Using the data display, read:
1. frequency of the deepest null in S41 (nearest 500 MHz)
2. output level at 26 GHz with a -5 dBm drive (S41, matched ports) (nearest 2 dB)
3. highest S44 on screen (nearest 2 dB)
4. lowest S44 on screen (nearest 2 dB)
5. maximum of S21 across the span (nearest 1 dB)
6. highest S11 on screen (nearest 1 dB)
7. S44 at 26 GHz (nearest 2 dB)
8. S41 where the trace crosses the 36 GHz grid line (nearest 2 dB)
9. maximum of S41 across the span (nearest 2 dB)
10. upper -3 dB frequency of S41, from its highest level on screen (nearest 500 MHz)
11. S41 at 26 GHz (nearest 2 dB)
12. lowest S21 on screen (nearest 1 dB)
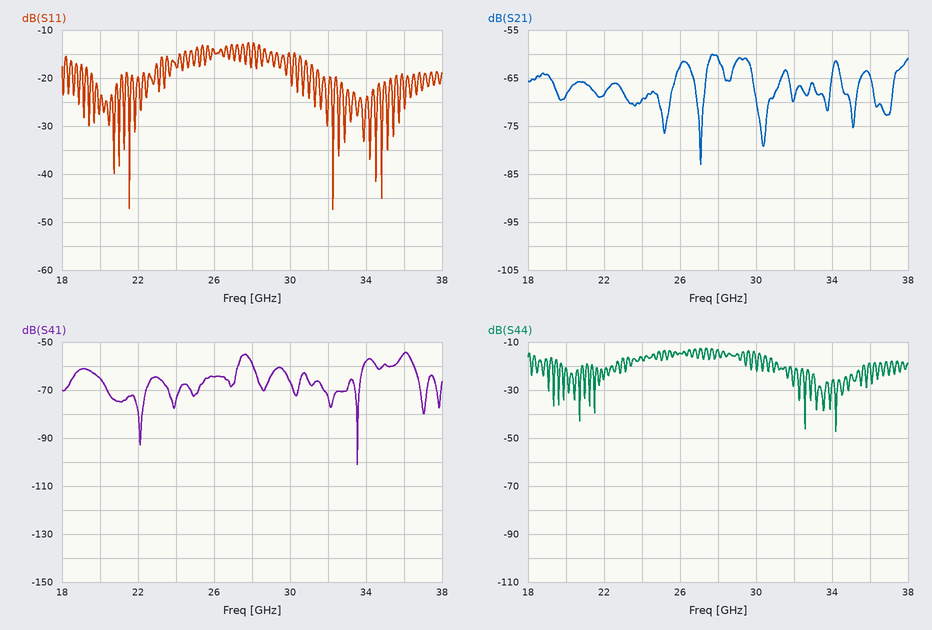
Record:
33.5 GHz
-70 dBm
-12 dB
-48 dB
-60 dB
-13 dB
-14 dB
-54 dB
-54 dB
36.5 GHz
-64 dB
-83 dB
